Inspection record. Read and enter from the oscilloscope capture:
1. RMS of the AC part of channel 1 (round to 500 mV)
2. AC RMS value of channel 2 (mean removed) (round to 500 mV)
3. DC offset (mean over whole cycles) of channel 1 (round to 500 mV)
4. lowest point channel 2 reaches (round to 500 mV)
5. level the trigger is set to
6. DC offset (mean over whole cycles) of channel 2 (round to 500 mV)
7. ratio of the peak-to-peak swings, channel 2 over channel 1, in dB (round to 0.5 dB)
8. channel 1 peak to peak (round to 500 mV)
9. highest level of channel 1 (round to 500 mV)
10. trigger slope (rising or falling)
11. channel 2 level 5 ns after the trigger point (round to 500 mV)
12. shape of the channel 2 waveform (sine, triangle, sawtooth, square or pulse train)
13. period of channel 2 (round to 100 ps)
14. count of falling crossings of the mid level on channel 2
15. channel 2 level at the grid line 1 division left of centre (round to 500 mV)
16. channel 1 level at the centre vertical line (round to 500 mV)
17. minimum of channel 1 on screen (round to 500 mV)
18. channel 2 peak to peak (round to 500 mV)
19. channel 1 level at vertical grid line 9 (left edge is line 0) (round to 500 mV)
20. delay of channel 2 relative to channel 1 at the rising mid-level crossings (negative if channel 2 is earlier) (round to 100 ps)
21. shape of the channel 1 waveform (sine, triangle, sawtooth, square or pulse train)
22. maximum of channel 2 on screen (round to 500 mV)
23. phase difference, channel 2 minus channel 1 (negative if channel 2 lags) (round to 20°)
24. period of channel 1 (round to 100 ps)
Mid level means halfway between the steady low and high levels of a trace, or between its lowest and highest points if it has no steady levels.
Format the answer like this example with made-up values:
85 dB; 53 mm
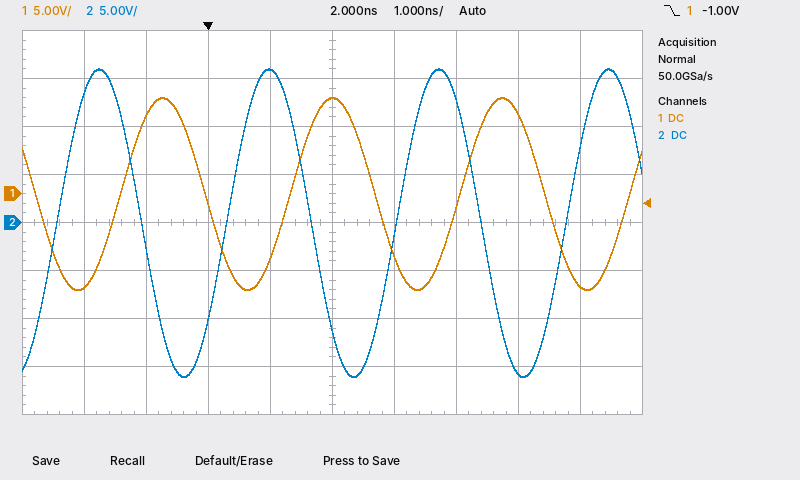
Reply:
7.0 V; 11.5 V; 0.0 V; -16.0 V; -1.00 V; 0.0 V; 4.0 dB; 20.0 V; 10.0 V; falling; -15.5 V; sine; 2.7 ns; 3; 16.0 V; 10.0 V; -10.0 V; 32.0 V; -9.5 V; -1.0 ns; sine; 16.0 V; +140°; 2.7 ns
